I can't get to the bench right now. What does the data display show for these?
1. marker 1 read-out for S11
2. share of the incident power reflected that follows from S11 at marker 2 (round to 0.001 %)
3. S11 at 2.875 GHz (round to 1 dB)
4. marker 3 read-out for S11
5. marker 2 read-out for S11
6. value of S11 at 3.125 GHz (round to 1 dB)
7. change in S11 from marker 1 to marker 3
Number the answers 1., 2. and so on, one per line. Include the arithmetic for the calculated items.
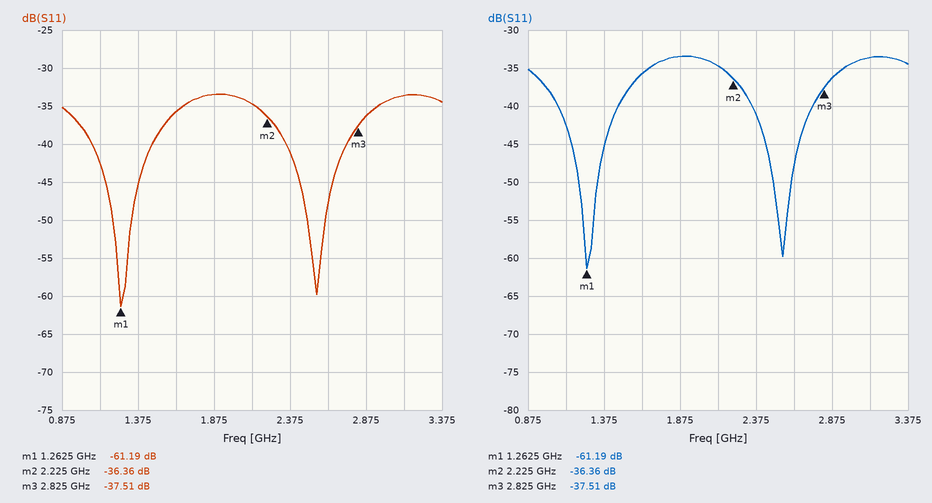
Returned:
1. -61.19 dB
2. 10^(-36.36/10) ≈ 0.023 %
3. -36 dB
4. -37.51 dB
5. -36.36 dB
6. -34 dB
7. -37.51 − (-61.19) = 23.68 dB
